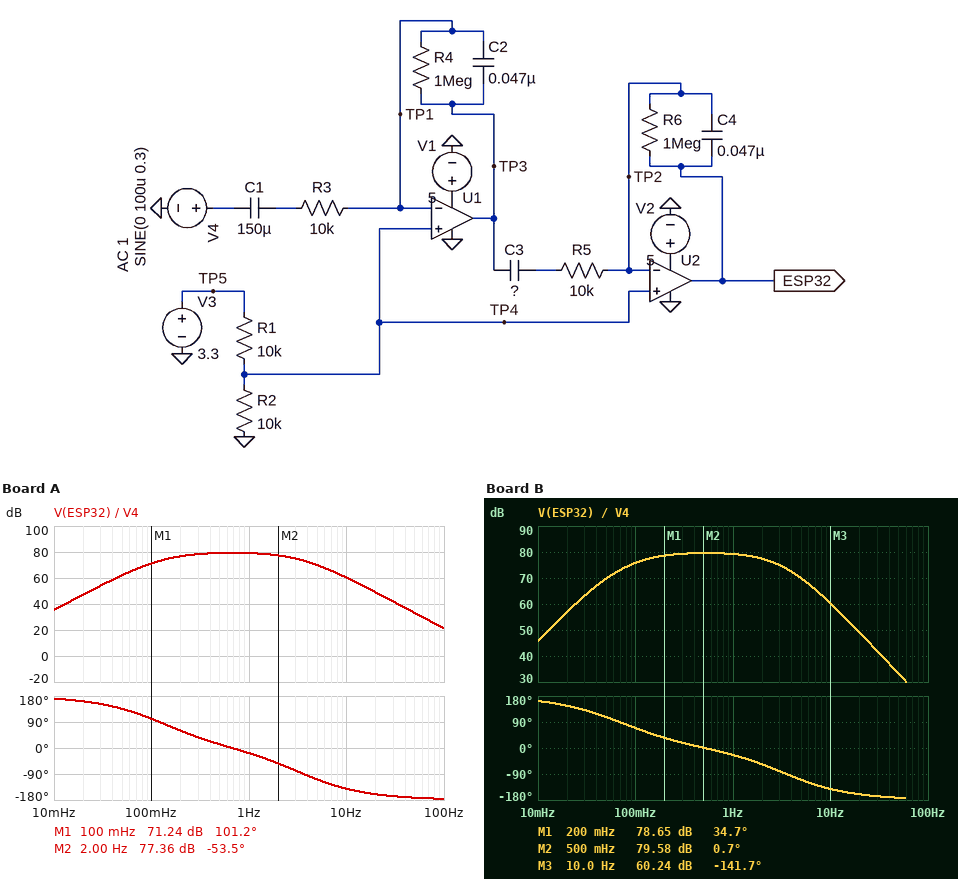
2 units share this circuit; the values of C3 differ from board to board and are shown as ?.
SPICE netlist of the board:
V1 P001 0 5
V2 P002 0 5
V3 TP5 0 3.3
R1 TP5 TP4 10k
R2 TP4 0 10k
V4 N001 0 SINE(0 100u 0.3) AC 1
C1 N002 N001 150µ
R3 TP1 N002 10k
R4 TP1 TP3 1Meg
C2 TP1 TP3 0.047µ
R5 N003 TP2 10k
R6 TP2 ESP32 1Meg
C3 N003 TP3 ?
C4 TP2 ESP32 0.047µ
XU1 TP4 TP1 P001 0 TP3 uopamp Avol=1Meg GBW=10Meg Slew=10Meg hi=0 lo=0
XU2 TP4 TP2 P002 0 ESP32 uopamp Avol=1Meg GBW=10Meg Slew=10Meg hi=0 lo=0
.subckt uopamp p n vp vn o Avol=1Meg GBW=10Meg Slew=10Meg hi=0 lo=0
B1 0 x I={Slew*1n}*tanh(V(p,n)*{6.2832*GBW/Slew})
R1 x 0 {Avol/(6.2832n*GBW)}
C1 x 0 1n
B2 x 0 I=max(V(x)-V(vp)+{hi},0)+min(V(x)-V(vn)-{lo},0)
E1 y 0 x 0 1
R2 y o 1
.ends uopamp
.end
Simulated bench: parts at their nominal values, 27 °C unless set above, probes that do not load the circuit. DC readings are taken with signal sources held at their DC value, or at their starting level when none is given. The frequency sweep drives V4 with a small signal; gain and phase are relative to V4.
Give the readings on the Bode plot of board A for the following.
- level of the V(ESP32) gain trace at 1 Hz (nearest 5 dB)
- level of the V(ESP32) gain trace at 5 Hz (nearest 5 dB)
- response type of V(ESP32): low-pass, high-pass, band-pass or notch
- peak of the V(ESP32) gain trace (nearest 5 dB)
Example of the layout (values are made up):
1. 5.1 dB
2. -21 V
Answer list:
1. 80 dB
2. 70 dB
3. band-pass
4. 80 dB
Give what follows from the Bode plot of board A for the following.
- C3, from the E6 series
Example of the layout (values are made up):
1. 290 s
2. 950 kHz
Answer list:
1. 100 µF
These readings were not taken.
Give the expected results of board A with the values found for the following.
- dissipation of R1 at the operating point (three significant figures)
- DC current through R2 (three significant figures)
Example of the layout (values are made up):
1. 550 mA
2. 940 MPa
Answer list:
1. 272 µW
2. 165 µA
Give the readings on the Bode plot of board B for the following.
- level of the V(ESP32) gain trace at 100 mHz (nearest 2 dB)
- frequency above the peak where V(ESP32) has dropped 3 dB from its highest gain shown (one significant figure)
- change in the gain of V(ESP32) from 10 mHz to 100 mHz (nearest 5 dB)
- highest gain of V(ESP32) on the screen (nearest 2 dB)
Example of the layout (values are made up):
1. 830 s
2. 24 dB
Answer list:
1. 76 dB
2. 2 Hz
3. 30 dB
4. 80 dB
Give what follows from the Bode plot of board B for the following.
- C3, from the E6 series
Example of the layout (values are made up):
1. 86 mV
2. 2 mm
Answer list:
1. 330 µF
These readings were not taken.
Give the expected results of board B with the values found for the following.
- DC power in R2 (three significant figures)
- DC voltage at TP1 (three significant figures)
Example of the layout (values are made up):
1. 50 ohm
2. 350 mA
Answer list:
1. 272 µW
2. 1.65 V
